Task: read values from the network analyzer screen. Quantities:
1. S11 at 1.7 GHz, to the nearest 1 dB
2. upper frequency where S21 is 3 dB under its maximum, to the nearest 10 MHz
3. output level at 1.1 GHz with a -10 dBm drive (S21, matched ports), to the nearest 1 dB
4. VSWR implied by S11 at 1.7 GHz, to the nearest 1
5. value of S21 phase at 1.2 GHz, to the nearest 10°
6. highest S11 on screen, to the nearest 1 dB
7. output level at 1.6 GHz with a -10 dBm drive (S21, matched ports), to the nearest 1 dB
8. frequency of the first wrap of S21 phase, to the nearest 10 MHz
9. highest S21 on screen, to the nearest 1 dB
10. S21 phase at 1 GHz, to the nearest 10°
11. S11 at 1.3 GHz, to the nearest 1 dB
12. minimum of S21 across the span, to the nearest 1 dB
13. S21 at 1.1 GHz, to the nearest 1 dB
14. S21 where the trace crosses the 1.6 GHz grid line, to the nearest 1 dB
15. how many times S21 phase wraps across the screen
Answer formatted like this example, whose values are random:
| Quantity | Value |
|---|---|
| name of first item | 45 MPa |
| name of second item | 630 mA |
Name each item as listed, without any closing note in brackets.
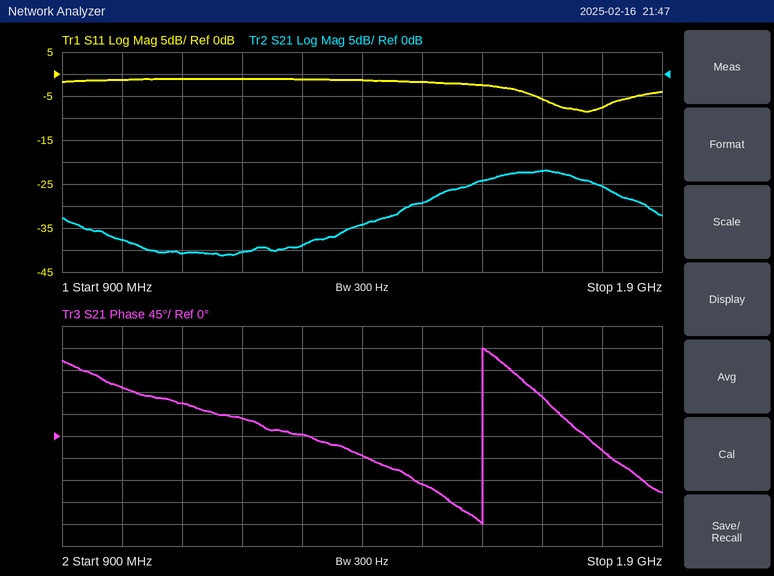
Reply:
| Quantity | Value |
|---|---|
| S11 at 1.7 GHz, to the nearest 1 dB | -6 dB |
| upper frequency where S21 is 3 dB under its maximum, to the nearest 10 MHz | 1.79 GHz |
| output level at 1.1 GHz with a -10 dBm drive (S21, matched ports), to the nearest 1 dB | -51 dBm |
| VSWR implied by S11 at 1.7 GHz, to the nearest 1 | 3 |
| value of S21 phase at 1.2 GHz, to the nearest 10° | 40° |
| highest S11 on screen, to the nearest 1 dB | -1 dB |
| output level at 1.6 GHz with a -10 dBm drive (S21, matched ports), to the nearest 1 dB | -34 dBm |
| frequency of the first wrap of S21 phase, to the nearest 10 MHz | 1.60 GHz |
| highest S21 on screen, to the nearest 1 dB | -22 dB |
| S21 phase at 1 GHz, to the nearest 10° | 100° |
| S11 at 1.3 GHz, to the nearest 1 dB | -1 dB |
| minimum of S21 across the span, to the nearest 1 dB | -41 dB |
| S21 at 1.1 GHz, to the nearest 1 dB | -41 dB |
| S21 where the trace crosses the 1.6 GHz grid line, to the nearest 1 dB | -24 dB |
| how many times S21 phase wraps across the screen | 1 |
